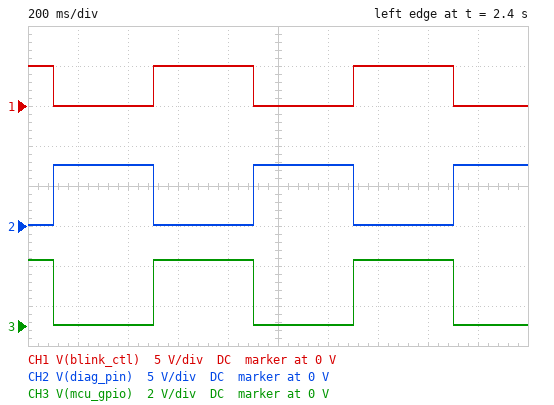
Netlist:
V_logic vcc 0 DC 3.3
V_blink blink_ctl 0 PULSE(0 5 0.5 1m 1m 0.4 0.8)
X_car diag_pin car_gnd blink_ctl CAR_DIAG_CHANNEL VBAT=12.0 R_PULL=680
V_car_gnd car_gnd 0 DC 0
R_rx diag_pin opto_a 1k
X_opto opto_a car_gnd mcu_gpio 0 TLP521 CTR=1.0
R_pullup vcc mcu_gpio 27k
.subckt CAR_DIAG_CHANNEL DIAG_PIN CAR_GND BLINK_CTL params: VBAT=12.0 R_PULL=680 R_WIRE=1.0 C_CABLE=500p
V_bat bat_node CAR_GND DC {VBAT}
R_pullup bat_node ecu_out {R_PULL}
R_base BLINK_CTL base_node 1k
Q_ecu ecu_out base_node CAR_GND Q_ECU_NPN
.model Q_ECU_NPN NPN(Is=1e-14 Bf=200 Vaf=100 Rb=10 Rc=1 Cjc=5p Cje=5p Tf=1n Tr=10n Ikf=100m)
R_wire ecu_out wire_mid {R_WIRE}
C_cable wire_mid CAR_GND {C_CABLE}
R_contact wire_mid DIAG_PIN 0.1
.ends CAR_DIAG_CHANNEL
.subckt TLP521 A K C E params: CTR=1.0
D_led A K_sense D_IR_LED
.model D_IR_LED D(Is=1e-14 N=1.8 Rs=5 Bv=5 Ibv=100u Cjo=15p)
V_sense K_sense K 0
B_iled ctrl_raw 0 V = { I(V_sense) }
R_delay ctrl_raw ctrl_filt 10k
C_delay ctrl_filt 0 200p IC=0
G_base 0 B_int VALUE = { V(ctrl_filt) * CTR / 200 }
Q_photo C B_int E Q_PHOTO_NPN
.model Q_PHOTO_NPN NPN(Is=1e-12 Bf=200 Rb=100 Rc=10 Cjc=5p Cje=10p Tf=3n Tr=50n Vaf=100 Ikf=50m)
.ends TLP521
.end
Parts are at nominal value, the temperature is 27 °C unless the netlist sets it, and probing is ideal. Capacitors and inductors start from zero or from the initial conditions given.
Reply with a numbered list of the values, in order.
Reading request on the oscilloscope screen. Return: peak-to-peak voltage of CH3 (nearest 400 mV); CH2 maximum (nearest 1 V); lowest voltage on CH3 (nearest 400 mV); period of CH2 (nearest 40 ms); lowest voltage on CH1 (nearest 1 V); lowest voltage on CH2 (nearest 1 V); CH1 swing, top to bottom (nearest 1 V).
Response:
1. 3.2 V
2. 8 V
3. 0 V
4. 800 ms
5. 0 V
6. 0 V
7. 5 V
